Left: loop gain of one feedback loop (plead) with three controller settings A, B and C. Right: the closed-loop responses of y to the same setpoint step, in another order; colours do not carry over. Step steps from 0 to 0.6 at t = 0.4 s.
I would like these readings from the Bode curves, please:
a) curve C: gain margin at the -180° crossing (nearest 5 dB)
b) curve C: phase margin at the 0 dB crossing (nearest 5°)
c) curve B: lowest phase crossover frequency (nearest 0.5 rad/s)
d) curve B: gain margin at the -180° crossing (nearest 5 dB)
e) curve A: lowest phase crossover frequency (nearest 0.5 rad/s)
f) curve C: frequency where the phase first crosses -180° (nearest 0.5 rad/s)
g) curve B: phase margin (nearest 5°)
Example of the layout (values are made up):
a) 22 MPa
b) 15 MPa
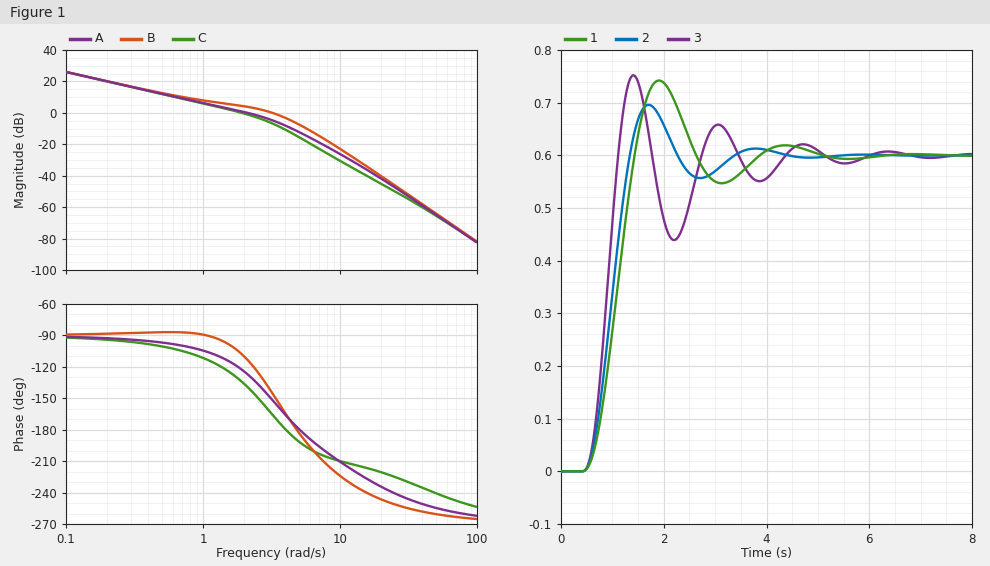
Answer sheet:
a) 10 dB
b) 45°
c) 5.0 rad/s
d) 5 dB
e) 5.0 rad/s
f) 4.0 rad/s
g) 35°
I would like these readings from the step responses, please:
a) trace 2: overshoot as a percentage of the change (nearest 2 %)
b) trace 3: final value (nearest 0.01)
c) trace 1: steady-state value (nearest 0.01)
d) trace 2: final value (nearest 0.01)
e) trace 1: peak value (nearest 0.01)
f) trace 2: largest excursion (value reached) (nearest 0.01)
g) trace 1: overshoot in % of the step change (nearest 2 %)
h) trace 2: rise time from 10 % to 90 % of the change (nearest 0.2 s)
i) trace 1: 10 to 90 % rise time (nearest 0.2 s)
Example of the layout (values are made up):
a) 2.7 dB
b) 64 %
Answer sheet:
a) 16 %
b) 0.60
c) 0.60
d) 0.60
e) 0.74
f) 0.70
g) 24 %
h) 0.6 s
i) 0.6 s
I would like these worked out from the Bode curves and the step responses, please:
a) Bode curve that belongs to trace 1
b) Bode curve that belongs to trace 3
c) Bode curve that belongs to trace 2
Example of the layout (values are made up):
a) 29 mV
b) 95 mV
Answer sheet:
a) C
b) B
c) A
